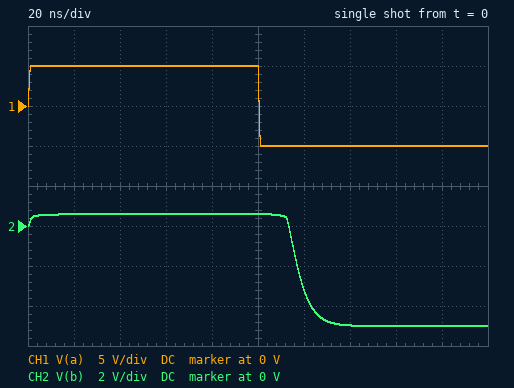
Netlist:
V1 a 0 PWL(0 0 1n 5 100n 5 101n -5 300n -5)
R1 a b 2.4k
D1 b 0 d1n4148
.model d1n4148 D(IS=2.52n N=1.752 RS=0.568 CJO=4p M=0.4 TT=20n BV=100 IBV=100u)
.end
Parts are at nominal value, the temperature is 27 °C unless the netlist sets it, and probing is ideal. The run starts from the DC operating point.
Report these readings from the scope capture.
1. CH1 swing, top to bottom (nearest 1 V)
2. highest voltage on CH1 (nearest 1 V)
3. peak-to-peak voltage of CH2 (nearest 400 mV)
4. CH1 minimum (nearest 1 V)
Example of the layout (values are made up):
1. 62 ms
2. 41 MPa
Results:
1. 10 V
2. 5 V
3. 5.6 V
4. -5 V
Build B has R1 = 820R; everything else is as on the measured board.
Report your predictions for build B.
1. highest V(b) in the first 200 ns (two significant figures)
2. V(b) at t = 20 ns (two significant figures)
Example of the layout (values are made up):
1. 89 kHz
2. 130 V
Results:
1. 660 mV
2. 640 mV
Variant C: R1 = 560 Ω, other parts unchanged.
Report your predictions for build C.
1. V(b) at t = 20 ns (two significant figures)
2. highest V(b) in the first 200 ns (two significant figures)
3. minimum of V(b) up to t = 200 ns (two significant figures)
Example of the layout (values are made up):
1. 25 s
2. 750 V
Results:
1. 660 mV
2. 680 mV
3. -5.0 V
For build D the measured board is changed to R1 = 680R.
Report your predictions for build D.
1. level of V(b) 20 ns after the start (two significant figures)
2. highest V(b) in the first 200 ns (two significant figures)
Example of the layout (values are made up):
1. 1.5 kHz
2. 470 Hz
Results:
1. 650 mV
2. 670 mV
